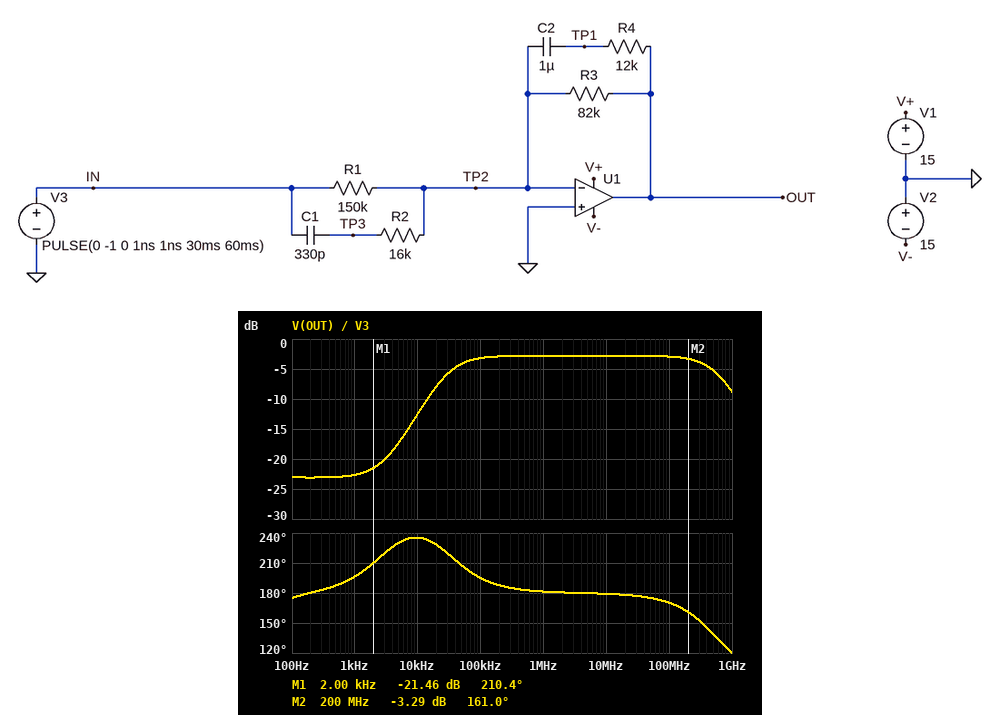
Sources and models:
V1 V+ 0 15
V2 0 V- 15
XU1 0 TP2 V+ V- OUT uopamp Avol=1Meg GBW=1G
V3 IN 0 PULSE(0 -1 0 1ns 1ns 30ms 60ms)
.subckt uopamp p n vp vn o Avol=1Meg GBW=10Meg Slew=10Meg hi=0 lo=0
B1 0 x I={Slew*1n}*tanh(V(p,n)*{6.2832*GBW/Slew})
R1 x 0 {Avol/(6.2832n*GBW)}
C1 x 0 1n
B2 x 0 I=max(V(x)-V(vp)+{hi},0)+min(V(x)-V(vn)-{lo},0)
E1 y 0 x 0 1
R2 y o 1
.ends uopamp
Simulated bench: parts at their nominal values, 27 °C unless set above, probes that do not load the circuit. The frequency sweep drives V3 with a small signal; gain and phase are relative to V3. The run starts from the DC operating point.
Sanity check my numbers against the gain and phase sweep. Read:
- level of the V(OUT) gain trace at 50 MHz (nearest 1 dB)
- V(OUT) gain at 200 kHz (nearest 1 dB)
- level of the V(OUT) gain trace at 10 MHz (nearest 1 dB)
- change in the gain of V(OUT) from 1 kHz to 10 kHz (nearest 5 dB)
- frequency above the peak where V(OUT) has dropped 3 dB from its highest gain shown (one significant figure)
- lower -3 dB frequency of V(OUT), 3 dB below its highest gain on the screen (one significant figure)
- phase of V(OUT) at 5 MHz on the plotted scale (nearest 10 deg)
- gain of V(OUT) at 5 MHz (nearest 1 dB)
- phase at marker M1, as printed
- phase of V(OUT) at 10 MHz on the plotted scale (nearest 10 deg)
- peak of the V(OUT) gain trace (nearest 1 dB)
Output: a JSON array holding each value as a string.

["-3 dB", "-3 dB", "-3 dB", "10 dB", "600 MHz", "30 kHz", "180 deg", "-3 dB", "210.4 deg", "180 deg", "-3 dB"]
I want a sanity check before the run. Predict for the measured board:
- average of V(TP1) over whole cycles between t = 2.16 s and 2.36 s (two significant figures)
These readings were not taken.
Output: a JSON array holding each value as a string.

["270 mV"]
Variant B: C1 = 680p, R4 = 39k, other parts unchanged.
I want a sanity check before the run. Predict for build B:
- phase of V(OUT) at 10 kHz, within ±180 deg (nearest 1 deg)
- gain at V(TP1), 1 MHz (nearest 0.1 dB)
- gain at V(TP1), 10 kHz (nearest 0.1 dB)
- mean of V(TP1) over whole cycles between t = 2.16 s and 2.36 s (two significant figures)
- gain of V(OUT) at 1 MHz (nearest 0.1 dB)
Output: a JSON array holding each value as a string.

["-132 deg", "-54.7 dB", "-67.2 dB", "270 mV", "5.2 dB"]
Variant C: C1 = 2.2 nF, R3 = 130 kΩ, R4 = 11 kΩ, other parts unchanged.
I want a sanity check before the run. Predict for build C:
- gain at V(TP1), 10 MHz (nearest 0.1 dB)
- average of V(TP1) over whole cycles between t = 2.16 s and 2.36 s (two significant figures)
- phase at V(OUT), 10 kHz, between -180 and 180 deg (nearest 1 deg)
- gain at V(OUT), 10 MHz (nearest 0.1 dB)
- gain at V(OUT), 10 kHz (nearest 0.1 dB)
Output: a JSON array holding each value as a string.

["-43.1 dB", "430 mV", "-158 deg", "-3.1 dB", "-3.9 dB"]
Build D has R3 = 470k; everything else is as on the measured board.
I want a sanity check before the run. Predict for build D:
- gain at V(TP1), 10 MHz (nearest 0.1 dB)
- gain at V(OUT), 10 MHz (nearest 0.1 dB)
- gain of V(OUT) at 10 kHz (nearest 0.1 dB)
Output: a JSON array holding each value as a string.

["-41.8 dB", "-1.8 dB", "-11.5 dB"]
